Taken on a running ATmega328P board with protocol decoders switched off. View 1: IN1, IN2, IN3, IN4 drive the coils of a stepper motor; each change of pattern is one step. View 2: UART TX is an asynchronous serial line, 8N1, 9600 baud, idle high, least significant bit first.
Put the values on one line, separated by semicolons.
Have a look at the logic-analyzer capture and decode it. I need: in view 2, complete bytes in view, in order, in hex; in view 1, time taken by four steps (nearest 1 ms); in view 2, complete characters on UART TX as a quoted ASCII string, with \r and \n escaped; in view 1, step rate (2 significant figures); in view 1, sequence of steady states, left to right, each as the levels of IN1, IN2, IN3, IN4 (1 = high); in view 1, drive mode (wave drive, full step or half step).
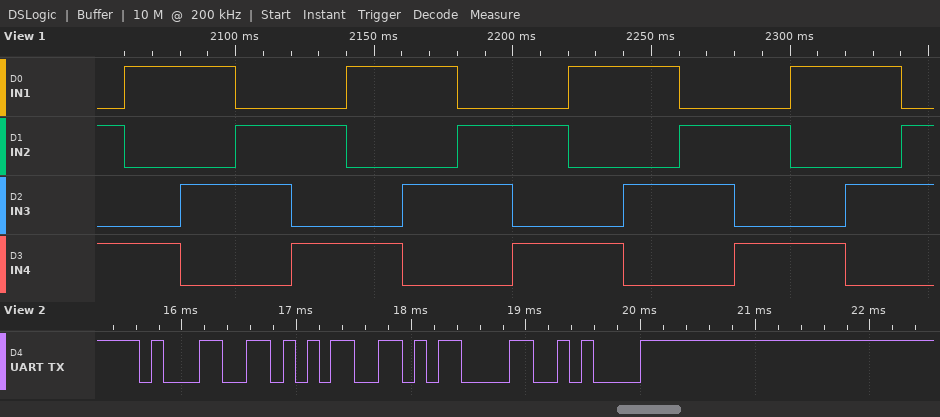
0x31 0x35 0x0D 0x0A; 80 ms; "15\r\n"; 50 steps/s; 0101 1001 1010 0110 0101 1001 1010 0110 0101 1001 1010 0110 0101 1001 1010 0110; full step
